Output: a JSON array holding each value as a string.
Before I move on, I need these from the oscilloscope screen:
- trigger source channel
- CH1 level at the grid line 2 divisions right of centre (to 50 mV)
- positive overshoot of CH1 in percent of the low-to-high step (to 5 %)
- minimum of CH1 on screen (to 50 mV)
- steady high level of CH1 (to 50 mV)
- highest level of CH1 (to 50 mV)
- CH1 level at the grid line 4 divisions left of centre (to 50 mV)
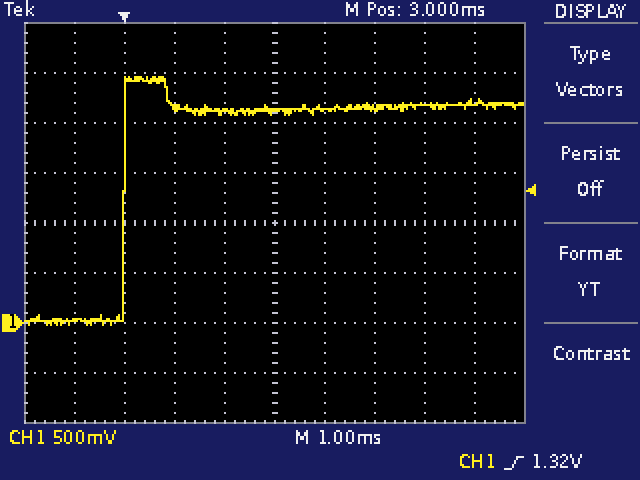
["CH1", "2.15 V", "15 %", "0 mV", "2.15 V", "2.45 V", "50 mV"]
